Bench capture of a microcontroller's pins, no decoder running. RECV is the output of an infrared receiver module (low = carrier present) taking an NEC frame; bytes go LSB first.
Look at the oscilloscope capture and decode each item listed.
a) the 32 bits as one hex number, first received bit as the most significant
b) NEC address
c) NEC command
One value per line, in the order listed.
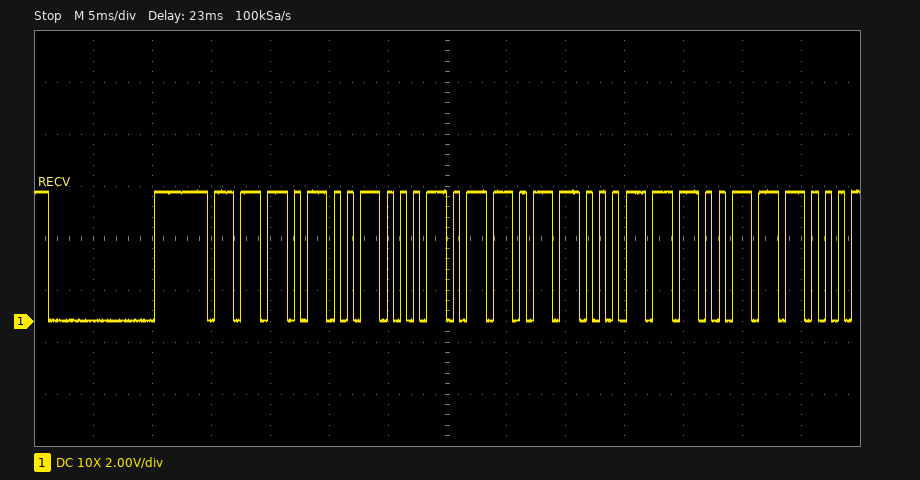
0xE916C738
0x97
0xE3
